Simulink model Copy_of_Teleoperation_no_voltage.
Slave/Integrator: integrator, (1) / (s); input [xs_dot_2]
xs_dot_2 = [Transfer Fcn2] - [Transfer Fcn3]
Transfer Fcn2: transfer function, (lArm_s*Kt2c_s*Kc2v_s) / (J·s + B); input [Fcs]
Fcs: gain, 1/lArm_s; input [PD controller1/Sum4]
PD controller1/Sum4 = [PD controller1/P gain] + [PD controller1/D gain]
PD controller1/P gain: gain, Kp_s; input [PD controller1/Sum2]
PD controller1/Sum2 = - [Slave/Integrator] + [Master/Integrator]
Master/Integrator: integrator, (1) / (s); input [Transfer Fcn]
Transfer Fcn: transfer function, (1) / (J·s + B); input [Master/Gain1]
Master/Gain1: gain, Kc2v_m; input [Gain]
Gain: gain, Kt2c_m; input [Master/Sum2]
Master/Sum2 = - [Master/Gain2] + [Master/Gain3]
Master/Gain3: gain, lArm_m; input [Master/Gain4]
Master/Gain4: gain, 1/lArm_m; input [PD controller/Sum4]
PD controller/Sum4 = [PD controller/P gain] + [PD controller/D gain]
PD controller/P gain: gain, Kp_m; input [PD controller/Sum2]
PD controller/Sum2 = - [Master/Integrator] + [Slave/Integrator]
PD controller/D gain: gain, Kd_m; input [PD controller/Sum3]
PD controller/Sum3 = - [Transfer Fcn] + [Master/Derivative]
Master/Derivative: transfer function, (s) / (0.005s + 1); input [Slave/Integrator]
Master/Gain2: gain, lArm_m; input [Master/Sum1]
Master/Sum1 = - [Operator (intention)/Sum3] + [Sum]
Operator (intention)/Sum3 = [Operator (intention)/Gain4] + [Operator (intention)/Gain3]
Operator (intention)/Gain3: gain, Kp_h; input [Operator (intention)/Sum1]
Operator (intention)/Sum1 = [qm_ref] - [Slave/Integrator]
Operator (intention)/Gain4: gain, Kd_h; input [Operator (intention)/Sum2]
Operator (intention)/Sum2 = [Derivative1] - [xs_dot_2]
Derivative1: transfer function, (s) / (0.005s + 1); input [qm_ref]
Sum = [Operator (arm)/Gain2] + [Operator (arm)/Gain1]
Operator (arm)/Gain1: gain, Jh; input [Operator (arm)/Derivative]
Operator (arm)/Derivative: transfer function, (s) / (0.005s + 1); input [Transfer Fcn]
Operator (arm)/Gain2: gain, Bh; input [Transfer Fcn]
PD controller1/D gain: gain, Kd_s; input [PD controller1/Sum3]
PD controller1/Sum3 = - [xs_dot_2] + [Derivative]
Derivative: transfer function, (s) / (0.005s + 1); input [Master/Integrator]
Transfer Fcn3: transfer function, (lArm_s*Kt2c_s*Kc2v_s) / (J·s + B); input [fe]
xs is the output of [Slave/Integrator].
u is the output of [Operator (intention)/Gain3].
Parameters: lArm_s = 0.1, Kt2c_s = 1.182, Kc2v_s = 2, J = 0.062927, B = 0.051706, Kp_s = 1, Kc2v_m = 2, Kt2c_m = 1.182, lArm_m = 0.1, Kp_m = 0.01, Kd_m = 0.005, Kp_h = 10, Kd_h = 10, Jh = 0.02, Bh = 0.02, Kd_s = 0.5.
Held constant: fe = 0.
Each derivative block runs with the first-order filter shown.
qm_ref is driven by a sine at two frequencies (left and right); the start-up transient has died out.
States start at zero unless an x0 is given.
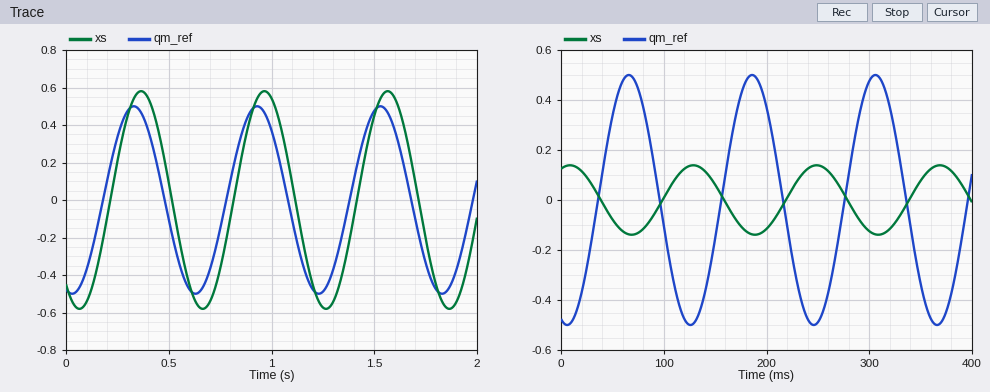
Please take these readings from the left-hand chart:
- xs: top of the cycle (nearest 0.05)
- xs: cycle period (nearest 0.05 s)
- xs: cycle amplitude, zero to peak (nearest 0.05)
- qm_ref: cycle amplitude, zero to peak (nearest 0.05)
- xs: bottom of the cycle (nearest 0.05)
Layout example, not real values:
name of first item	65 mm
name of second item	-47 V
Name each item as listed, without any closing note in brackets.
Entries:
xs: top of the cycle	0.60
xs: cycle period	0.60 s
xs: cycle amplitude, zero to peak	0.60
qm_ref: cycle amplitude, zero to peak	0.50
xs: bottom of the cycle	-0.60
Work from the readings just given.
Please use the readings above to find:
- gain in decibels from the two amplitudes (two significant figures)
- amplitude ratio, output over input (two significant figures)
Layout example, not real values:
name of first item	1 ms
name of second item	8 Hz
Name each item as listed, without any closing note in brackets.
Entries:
gain in decibels from the two amplitudes	1.6 dB
amplitude ratio, output over input	1.2
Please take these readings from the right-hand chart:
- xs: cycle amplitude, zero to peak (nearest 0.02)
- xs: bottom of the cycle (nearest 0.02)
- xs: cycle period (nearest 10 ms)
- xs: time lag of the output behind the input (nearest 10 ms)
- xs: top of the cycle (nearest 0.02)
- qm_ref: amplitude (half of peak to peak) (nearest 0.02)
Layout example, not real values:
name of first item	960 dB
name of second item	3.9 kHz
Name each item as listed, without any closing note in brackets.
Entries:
xs: cycle amplitude, zero to peak	0.14
xs: bottom of the cycle	-0.14
xs: cycle period	120 ms
xs: time lag of the output behind the input	60 ms
xs: top of the cycle	0.14
qm_ref: amplitude (half of peak to peak)	0.50
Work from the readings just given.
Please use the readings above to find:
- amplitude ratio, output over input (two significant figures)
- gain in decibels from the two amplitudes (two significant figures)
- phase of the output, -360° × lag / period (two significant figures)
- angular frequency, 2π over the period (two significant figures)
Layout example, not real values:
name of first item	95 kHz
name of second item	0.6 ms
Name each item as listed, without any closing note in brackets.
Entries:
amplitude ratio, output over input	0.28
gain in decibels from the two amplitudes	-11 dB
phase of the output, -360° × lag / period	-180°
angular frequency, 2π over the period	0.052 rad/ms
